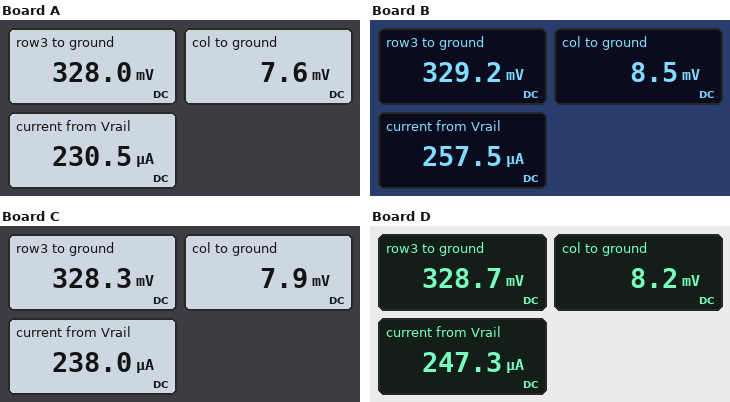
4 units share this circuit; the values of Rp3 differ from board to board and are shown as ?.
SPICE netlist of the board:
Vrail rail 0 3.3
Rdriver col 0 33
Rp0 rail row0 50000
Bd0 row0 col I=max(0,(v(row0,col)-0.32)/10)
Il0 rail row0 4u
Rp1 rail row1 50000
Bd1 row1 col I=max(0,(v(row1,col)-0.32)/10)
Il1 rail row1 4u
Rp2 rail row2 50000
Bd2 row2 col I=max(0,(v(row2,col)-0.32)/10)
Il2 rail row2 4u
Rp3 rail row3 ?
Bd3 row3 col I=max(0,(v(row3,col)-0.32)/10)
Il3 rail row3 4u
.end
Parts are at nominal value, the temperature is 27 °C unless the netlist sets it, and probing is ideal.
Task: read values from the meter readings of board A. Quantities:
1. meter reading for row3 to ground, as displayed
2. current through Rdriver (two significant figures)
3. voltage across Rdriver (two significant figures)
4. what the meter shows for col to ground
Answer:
328.0 mV
230 µA
7.6 mV
7.6 mV
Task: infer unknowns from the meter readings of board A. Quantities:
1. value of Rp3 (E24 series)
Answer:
82 kΩ
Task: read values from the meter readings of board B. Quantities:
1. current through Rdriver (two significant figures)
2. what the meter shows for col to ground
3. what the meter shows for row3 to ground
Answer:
260 µA
8.5 mV
329.2 mV
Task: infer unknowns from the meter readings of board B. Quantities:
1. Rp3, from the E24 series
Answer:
47 kΩ
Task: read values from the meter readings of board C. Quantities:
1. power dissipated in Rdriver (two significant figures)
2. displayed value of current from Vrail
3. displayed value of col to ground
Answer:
1.9 µW
238.0 µA
7.9 mV
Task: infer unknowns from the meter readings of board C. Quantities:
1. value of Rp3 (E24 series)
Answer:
68 kΩ
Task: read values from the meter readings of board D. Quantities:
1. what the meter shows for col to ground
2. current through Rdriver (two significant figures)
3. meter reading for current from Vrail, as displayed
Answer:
8.2 mV
250 µA
247.3 µA
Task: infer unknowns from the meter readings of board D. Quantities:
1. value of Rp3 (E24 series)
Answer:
56 kΩ
